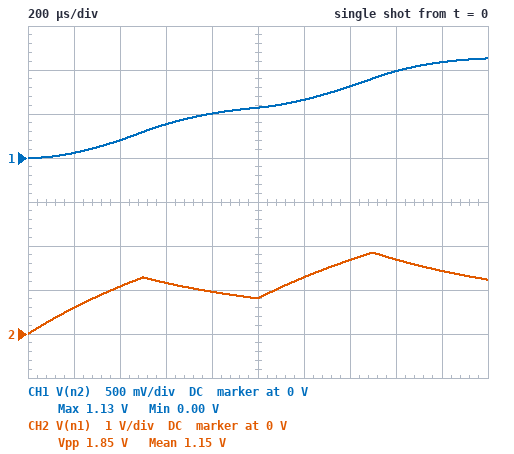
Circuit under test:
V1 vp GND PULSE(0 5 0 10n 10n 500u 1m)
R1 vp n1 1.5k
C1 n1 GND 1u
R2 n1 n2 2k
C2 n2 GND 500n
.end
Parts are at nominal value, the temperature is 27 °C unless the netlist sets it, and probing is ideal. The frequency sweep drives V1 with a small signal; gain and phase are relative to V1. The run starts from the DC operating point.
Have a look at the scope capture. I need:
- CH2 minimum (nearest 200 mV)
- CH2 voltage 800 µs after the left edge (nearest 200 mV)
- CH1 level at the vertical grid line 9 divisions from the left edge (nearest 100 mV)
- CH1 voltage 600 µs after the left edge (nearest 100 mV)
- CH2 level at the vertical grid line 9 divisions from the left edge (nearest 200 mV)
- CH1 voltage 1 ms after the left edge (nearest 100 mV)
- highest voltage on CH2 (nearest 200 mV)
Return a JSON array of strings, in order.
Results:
["0 V", "1.0 V", "1.1 V", "400 mV", "1.4 V", "600 mV", "1.8 V"]
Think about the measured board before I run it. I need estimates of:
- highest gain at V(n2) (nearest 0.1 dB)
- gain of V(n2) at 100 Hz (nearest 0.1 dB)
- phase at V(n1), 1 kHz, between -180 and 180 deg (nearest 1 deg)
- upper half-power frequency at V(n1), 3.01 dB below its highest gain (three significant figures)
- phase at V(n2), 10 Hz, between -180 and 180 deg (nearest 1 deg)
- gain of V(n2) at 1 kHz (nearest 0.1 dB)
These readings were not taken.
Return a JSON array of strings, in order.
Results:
["0 dB", "-6.4 dB", "-80 deg", "65.3 Hz", "-12 deg", "-35.8 dB"]
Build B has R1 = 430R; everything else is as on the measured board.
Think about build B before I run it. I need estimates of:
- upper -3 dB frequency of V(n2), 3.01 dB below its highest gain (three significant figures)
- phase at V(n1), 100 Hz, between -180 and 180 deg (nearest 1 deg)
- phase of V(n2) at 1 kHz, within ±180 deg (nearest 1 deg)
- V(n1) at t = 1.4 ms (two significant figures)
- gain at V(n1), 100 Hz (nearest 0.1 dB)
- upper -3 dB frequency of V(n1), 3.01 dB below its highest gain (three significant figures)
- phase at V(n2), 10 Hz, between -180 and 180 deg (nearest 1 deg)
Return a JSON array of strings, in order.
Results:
["114 Hz", "-19 deg", "-147 deg", "3.2 V", "-1.0 dB", "265 Hz", "-6 deg"]
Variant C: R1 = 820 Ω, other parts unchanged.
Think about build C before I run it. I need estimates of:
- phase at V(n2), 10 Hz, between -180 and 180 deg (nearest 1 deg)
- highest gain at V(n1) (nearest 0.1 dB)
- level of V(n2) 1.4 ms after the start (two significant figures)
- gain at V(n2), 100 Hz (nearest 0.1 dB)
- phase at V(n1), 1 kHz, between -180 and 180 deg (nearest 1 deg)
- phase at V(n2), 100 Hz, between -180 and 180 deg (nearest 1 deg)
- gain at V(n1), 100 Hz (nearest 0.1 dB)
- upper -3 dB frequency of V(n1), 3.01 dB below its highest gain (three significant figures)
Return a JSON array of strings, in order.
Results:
["-8 deg", "0 dB", "1.2 V", "-3.8 dB", "-75 deg", "-64 deg", "-2.4 dB", "121 Hz"]
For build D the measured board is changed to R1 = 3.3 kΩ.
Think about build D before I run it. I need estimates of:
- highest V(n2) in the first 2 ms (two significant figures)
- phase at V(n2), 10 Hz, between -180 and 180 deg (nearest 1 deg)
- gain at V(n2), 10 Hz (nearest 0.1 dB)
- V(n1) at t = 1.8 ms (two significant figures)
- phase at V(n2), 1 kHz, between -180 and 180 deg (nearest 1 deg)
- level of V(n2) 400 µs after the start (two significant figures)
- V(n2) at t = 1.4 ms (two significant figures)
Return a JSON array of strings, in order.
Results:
["650 mV", "-21 deg", "-0.5 dB", "880 mV", "-164 deg", "96 mV", "440 mV"]
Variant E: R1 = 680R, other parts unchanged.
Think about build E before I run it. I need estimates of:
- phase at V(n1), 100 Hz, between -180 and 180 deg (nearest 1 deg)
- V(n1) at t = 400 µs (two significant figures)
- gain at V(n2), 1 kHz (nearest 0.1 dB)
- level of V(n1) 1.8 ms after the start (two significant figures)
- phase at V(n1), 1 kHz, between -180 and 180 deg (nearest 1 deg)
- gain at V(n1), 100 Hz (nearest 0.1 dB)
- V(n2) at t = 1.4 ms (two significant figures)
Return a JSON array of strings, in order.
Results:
["-28 deg", "2.1 V", "-29.2 dB", "1.8 V", "-73 deg", "-1.9 dB", "1.3 V"]
